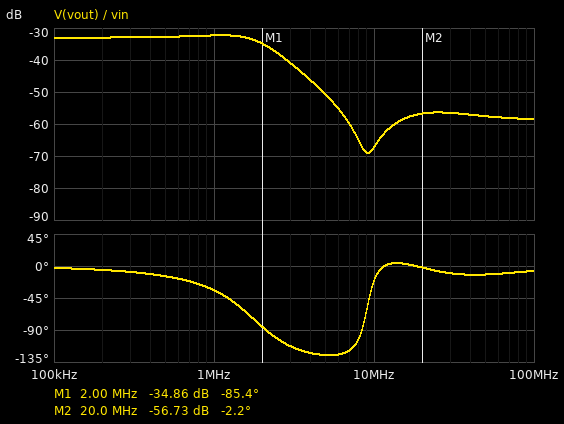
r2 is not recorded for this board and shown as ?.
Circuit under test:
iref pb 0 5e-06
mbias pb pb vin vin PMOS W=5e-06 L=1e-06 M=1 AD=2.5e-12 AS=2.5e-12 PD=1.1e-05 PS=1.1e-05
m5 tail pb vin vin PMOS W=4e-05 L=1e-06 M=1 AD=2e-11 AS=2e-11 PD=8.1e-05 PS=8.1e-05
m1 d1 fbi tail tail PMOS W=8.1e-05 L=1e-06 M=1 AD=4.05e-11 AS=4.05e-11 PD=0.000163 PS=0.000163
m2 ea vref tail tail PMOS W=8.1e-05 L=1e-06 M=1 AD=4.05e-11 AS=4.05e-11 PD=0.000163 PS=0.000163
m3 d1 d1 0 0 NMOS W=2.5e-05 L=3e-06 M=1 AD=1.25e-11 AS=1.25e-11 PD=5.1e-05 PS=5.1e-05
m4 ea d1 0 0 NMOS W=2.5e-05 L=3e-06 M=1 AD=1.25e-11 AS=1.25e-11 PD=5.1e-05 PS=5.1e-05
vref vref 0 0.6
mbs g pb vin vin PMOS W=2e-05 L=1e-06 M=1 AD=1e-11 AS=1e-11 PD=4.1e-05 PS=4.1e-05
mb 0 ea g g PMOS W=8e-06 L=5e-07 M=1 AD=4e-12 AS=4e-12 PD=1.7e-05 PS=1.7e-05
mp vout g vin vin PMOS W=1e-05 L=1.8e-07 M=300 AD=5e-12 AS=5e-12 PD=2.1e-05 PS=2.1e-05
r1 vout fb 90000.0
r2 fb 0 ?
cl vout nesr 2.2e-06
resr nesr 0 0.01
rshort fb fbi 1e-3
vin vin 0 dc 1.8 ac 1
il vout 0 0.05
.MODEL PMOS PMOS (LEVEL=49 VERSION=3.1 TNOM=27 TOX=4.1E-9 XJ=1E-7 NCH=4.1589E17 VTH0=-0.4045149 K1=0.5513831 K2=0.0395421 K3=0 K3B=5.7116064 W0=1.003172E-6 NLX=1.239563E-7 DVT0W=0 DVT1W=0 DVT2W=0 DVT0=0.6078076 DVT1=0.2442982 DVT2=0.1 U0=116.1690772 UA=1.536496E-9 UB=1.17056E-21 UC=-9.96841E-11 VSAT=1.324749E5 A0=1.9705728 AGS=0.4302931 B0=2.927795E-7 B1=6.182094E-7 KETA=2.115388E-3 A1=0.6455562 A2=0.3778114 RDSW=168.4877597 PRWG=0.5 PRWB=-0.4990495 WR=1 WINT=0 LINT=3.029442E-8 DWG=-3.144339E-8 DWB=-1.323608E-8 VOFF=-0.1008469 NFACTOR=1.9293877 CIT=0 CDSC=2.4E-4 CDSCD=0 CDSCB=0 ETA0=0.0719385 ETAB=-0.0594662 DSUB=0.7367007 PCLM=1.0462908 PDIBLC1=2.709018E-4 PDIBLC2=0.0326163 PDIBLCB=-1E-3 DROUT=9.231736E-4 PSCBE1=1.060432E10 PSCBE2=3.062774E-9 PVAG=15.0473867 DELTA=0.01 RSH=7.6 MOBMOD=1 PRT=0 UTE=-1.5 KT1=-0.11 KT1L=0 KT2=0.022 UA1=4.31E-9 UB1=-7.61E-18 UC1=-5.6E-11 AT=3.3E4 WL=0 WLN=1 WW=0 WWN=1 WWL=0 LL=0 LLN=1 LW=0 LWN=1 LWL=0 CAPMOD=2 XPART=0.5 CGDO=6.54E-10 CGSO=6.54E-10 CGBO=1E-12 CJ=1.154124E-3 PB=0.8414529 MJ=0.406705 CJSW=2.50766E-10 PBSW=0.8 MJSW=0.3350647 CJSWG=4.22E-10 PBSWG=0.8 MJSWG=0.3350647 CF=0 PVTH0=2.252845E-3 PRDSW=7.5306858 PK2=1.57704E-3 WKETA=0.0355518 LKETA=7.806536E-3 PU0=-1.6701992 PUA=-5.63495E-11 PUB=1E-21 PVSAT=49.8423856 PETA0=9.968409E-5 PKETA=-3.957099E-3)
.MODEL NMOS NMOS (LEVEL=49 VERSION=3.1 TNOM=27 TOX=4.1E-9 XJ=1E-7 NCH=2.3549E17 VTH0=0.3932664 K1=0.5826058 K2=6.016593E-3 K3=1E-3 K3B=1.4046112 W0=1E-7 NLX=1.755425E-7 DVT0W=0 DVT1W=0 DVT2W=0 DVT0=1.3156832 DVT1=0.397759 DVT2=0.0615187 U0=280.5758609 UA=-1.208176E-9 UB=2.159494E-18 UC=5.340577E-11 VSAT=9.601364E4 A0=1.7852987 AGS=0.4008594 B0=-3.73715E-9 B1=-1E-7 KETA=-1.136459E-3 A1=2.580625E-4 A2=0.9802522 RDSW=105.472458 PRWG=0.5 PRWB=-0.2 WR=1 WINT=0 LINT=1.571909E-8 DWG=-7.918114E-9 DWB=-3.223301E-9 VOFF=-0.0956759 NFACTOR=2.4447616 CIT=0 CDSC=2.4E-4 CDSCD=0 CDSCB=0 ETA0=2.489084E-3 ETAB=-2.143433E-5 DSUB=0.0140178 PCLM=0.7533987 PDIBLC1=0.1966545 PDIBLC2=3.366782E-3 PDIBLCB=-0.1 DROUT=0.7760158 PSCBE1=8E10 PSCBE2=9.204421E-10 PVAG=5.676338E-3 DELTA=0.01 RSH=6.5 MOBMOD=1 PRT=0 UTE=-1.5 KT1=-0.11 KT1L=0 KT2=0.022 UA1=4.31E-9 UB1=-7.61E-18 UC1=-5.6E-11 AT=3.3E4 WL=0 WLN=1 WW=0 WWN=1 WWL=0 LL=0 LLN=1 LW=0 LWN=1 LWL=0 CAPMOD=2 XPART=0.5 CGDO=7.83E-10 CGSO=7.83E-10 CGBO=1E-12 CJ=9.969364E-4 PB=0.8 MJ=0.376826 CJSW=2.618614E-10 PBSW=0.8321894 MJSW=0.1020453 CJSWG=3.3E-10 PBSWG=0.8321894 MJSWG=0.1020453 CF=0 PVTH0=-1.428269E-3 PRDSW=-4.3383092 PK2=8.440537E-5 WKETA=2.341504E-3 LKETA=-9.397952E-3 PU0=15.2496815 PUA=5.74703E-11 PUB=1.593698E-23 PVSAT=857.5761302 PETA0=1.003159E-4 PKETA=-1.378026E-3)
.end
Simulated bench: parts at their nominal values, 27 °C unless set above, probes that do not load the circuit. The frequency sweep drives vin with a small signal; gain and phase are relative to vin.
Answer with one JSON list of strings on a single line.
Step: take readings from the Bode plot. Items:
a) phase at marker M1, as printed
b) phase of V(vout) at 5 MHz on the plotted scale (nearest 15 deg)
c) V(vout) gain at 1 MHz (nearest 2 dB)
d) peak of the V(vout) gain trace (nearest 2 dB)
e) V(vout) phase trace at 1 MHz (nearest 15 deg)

["-85.4 deg", "-120 deg", "-32 dB", "-32 dB", "-30 deg"]
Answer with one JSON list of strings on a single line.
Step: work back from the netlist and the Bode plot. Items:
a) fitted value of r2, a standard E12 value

["82 kΩ"]
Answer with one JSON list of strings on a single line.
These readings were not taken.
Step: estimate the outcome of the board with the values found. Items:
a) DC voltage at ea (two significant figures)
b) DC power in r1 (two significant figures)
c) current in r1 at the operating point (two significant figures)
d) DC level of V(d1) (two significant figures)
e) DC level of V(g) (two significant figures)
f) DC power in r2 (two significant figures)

["390 mV", "4.8 µW", "7.3 µA", "560 mV", "1.0 V", "4.4 µW"]
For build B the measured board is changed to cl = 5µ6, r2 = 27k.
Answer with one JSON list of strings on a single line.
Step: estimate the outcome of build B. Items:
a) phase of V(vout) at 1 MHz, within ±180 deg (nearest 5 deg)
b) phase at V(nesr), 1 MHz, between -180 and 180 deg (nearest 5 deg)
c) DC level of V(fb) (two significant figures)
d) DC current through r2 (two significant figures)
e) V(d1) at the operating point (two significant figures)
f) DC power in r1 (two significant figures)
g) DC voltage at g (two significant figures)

["-70 deg", "0 deg", "400 mV", "15 µA", "620 mV", "20 µW", "660 mV"]
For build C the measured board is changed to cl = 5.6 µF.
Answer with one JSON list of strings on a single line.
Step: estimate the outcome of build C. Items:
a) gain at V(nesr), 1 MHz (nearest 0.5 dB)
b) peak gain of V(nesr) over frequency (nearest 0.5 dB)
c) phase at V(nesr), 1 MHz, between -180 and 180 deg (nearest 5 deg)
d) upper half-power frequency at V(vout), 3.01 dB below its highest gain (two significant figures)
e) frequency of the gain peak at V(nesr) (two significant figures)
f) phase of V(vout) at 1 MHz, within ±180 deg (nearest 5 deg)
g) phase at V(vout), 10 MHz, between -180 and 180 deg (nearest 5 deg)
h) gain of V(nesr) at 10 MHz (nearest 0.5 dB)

["-49.0 dB", "-48.5 dB", "10 deg", "530 kHz", "1.5 MHz", "-60 deg", "0 deg", "-69.0 dB"]
